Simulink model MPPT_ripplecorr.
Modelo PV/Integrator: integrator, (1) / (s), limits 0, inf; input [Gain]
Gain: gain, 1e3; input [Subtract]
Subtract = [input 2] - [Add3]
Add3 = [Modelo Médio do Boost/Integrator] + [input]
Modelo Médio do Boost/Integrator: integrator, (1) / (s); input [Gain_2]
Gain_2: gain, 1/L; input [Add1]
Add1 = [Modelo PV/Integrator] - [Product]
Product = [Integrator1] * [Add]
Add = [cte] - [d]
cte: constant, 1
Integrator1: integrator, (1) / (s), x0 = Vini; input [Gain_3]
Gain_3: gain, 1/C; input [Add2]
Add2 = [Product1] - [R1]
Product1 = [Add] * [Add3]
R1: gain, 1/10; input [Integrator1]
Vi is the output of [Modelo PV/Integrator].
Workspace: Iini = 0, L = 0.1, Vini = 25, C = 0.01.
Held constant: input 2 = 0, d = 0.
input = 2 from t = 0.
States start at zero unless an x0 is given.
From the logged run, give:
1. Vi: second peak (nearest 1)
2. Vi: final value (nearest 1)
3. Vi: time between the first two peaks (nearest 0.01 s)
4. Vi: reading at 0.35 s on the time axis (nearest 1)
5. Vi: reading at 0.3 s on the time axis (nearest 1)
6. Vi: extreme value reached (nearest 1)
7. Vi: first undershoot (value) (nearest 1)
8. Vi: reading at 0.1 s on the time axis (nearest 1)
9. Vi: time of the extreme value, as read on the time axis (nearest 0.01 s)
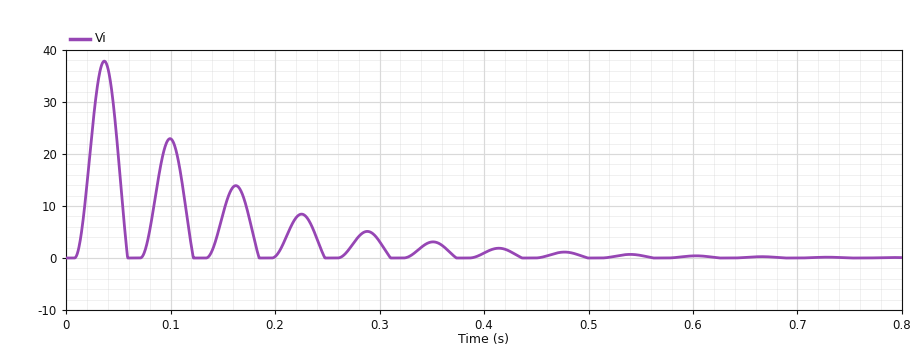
23
0
0.06 s
3
3
38
0
23
0.04 s
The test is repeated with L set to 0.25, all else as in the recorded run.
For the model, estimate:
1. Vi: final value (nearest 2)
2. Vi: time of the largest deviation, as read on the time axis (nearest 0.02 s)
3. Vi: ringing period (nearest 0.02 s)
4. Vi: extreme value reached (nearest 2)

0
0.06 s
0.10 s
32
